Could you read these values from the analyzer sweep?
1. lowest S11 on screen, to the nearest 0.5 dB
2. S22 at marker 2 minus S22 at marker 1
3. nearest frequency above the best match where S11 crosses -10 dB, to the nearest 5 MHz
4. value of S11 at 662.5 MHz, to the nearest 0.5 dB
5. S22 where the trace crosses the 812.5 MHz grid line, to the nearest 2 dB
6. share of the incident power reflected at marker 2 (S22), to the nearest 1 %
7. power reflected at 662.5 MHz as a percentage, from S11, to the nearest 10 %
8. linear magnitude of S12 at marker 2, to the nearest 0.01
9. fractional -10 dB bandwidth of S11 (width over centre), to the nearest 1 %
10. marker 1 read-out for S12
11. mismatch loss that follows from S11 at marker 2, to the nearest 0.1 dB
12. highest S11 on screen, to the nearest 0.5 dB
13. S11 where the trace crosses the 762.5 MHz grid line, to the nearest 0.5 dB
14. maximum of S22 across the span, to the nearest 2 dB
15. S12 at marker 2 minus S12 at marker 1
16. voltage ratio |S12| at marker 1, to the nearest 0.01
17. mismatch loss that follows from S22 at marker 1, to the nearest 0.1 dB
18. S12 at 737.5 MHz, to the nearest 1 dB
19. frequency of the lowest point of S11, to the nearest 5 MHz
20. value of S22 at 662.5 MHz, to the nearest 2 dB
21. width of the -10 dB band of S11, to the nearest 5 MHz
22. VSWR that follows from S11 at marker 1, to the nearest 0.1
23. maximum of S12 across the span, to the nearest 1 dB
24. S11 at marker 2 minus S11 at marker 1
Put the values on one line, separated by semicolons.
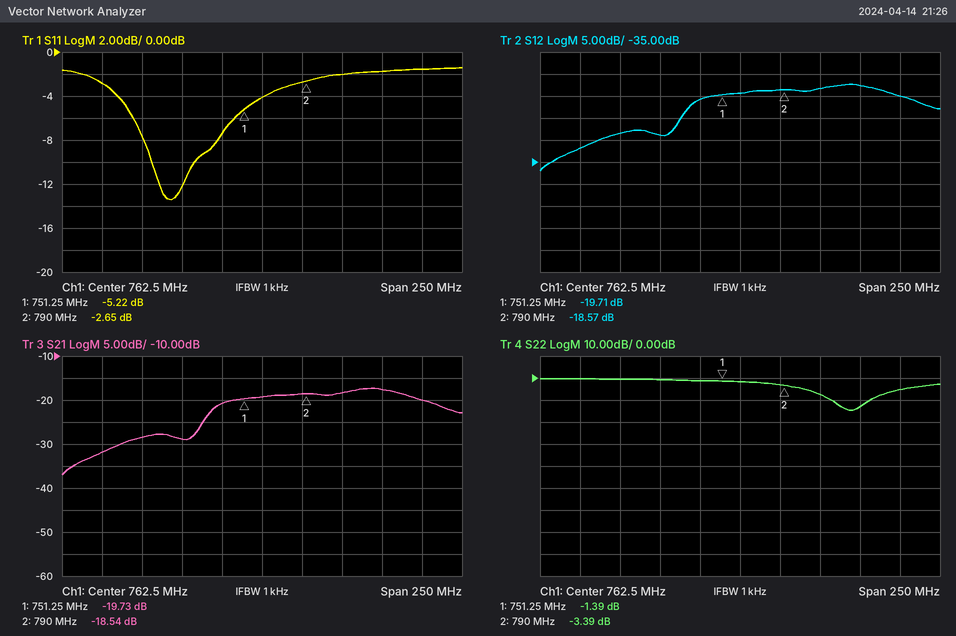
-13.5 dB; -2.00 dB; 720 MHz; -3.0 dB; -8 dB; 46 %; 50 %; 0.12; 4 %; -19.71 dB; 3.4 dB; -1.5 dB; -4.0 dB; 0 dB; 1.14 dB; 0.10; 5.6 dB; -21 dB; 705 MHz; 0 dB; 25 MHz; 3.4; -17 dB; 2.57 dB
